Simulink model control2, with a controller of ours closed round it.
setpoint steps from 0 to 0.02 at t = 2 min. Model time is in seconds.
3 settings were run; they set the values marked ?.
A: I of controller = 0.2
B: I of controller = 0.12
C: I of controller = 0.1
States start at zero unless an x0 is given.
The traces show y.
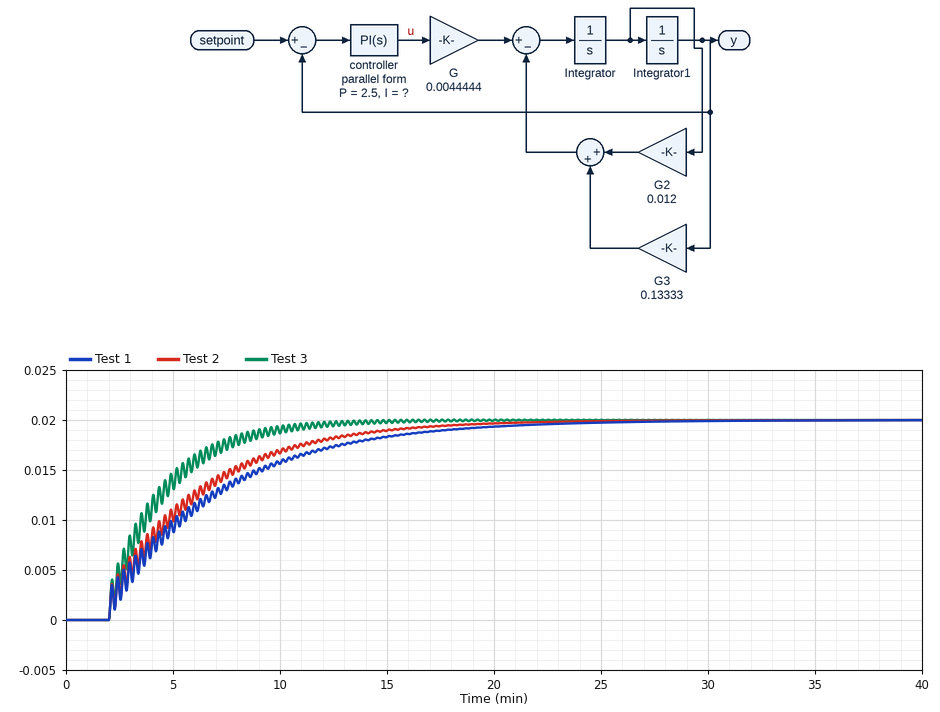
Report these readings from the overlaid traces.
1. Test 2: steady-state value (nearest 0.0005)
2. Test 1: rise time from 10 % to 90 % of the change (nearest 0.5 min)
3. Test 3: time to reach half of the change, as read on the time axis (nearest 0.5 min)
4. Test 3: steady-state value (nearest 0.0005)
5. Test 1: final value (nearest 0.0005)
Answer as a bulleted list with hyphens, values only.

- 0.0200
- 12.0 min
- 3.5 min
- 0.0200
- 0.0200
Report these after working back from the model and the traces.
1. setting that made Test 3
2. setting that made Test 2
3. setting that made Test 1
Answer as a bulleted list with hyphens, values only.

- A
- B
- C
